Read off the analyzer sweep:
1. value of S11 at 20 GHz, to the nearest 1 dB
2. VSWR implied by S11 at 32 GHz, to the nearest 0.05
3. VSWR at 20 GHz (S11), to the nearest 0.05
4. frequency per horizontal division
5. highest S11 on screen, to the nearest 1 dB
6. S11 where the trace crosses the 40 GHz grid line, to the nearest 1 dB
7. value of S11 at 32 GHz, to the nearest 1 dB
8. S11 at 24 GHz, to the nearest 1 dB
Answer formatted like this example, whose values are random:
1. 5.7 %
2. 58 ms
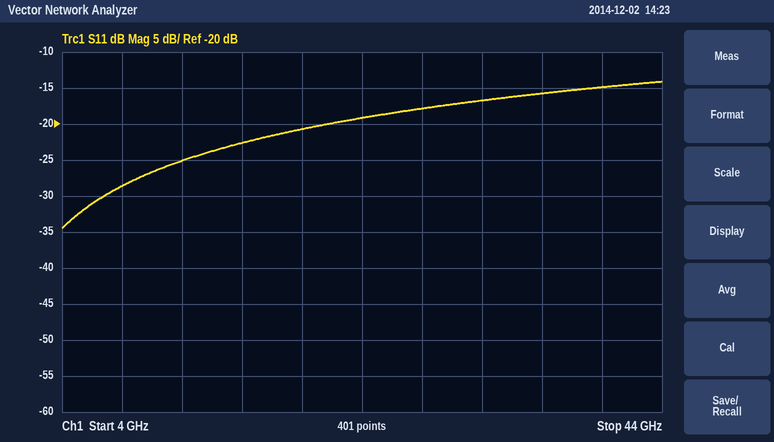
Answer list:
1. -21 dB
2. 1.35
3. 1.20
4. 4 GHz
5. -14 dB
6. -15 dB
7. -17 dB
8. -19 dB
